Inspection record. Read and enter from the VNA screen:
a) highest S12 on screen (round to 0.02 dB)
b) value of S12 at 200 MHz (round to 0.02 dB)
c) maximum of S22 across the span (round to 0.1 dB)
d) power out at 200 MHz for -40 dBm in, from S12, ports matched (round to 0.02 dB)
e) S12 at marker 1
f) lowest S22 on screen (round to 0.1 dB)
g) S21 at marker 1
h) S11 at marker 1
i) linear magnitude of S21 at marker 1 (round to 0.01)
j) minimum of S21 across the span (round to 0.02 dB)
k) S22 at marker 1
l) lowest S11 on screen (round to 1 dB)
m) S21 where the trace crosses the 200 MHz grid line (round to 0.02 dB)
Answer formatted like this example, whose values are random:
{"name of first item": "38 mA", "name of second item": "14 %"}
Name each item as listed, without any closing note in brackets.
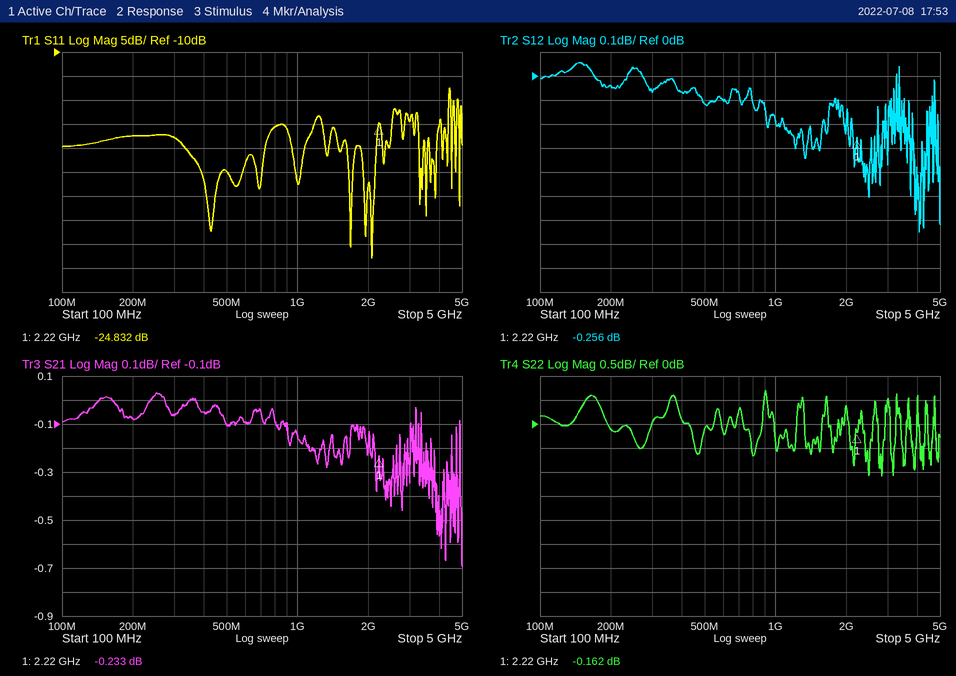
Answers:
{"highest S12 on screen": "0.06 dB", "value of S12 at 200 MHz": "-0.04 dB", "maximum of S22 across the span": "0.7 dB", "power out at 200 MHz for -40 dBm in, from S12, ports matched": "-40.04 dBm", "S12 at marker 1": "-0.256 dB", "lowest S22 on screen": "-1.1 dB", "S21 at marker 1": "-0.233 dB", "S11 at marker 1": "-24.832 dB", "linear magnitude of S21 at marker 1": "0.97", "minimum of S21 across the span": "-0.70 dB", "S22 at marker 1": "-0.162 dB", "lowest S11 on screen": "-53 dB", "S21 where the trace crosses the 200 MHz grid line": "-0.08 dB"}
